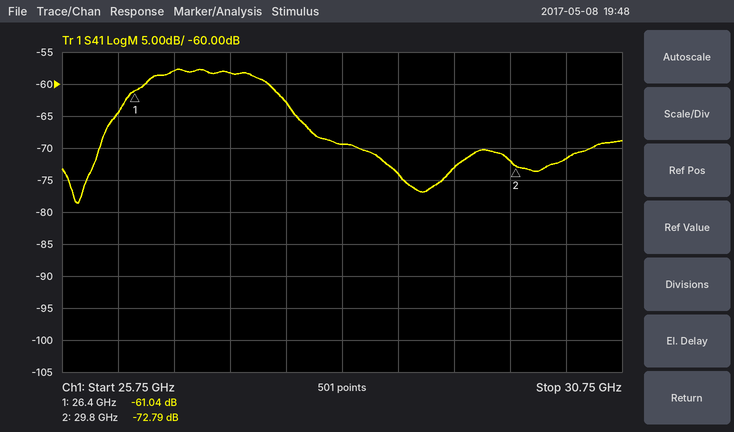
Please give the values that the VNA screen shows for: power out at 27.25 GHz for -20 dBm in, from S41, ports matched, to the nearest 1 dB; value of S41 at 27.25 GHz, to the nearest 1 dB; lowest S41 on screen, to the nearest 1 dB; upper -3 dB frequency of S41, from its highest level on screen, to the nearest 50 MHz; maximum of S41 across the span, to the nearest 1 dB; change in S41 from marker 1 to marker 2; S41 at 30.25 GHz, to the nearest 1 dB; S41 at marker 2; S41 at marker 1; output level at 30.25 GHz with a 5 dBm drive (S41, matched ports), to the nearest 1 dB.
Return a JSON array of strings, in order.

["-78 dBm", "-58 dB", "-79 dB", "27.65 GHz", "-58 dB", "-11.75 dB", "-72 dB", "-72.79 dB", "-61.04 dB", "-67 dBm"]
